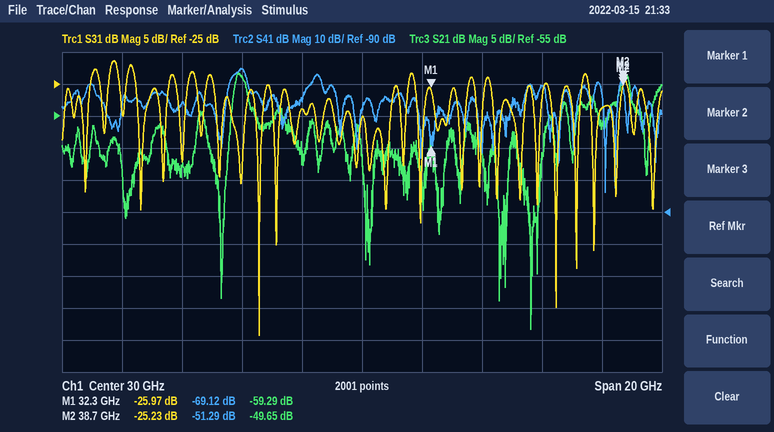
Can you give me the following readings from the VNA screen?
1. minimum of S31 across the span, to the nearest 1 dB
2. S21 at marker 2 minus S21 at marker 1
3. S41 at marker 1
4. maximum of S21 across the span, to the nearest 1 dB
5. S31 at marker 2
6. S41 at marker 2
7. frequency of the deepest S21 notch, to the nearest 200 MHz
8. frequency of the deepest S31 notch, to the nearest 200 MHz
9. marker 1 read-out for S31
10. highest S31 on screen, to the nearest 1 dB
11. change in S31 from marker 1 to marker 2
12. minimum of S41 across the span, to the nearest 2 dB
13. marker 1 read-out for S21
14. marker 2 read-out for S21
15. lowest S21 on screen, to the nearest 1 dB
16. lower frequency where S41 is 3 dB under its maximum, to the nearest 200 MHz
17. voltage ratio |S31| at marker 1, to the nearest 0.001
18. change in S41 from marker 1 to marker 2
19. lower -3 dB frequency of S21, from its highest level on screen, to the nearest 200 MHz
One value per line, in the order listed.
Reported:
-64 dB
9.64 dB
-69.12 dB
-48 dB
-25.23 dB
-51.29 dB
35.6 GHz
26.6 GHz
-25.97 dB
-21 dB
0.74 dB
-84 dB
-59.29 dB
-49.65 dB
-88 dB
25.6 GHz
0.050
17.83 dB
25.8 GHz
